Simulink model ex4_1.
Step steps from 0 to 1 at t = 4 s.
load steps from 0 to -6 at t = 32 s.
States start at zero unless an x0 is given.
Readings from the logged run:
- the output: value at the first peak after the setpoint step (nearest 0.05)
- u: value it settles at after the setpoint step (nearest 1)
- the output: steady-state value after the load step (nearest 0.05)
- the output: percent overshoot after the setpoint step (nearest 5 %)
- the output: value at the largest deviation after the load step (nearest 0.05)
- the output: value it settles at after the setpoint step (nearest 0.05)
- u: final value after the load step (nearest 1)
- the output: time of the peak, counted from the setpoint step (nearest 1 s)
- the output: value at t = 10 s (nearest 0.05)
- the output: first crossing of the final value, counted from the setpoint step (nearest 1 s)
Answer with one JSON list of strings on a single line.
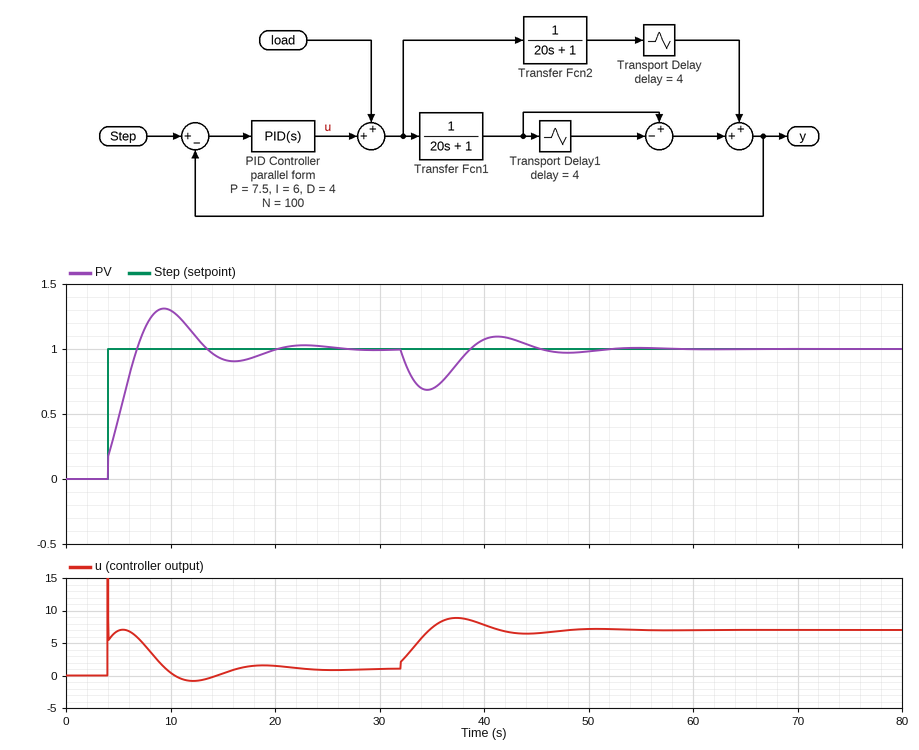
["1.30", "1", "1.00", "30 %", "0.70", "1.00", "7", "5 s", "1.30", "3 s"]
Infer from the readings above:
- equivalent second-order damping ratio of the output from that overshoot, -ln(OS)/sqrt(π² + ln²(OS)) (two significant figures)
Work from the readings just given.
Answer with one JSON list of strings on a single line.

["0.36"]
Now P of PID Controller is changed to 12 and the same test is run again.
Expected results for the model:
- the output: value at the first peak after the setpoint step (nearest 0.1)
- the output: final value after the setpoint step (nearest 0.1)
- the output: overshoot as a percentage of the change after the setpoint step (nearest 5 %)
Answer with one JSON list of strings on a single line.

["1.2", "1.0", "20 %"]
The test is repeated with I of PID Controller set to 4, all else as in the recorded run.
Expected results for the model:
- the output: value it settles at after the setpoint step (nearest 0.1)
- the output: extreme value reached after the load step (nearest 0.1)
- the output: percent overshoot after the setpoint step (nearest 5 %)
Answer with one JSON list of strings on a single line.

["1.0", "0.6", "25 %"]
